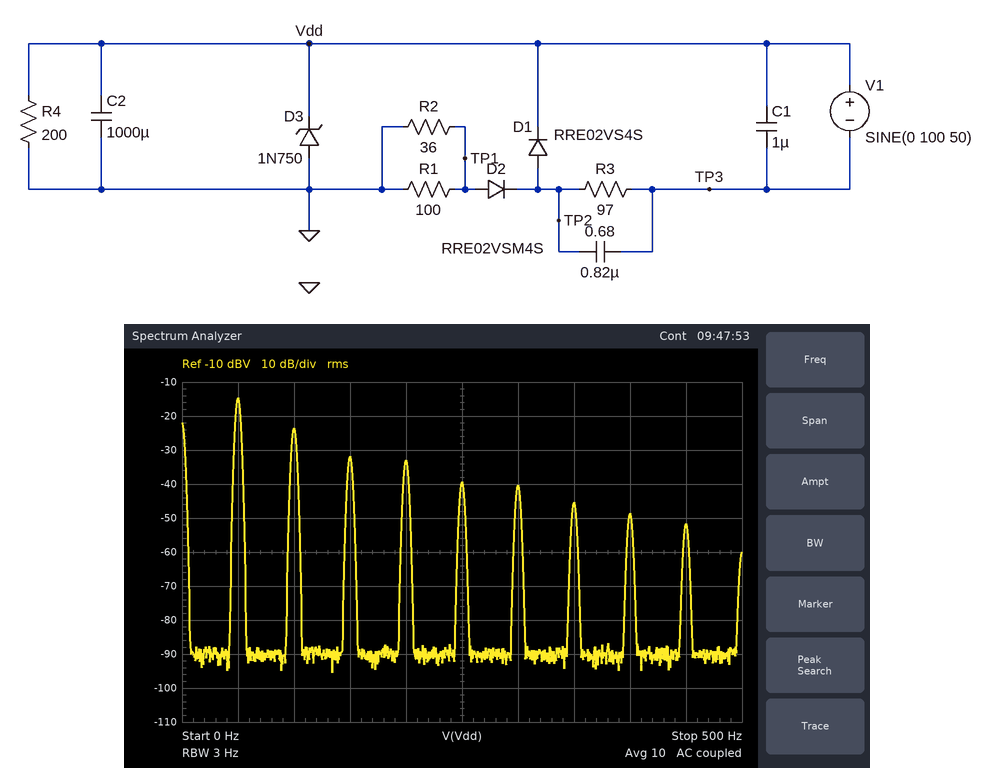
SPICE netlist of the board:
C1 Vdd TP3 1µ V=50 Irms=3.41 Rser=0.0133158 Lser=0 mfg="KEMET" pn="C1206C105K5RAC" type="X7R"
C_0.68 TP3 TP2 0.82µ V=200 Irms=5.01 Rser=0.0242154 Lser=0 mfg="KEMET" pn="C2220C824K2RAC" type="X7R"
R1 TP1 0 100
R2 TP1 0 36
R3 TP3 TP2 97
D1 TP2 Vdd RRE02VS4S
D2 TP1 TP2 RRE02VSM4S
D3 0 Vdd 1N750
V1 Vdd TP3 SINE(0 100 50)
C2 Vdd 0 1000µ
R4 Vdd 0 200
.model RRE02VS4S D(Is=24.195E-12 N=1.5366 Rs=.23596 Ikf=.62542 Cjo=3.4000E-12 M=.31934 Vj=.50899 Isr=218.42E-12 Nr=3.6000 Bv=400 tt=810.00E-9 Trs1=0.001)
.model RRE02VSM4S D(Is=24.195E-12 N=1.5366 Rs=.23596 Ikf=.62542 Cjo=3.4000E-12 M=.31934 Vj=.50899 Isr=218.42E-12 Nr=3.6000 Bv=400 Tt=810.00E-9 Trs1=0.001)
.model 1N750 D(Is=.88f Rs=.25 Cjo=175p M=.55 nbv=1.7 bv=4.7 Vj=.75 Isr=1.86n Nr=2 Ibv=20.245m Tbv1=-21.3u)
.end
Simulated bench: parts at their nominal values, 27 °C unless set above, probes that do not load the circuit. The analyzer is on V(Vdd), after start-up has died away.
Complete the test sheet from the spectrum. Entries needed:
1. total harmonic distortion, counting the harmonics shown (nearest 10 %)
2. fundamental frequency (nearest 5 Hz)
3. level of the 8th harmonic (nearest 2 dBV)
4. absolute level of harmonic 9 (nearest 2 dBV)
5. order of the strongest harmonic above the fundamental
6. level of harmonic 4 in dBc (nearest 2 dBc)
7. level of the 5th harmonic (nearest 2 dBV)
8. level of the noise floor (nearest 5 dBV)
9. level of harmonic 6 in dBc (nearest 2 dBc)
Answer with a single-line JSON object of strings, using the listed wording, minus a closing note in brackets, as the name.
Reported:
{"total harmonic distortion, counting the harmonics shown": "40 %", "fundamental frequency": "50 Hz", "level of the 8th harmonic": "-48 dBV", "absolute level of harmonic 9": "-52 dBV", "order of the strongest harmonic above the fundamental": "2", "level of harmonic 4 in dBc": "-18 dBc", "level of the 5th harmonic": "-40 dBV", "level of the noise floor": "-90 dBV", "level of harmonic 6 in dBc": "-26 dBc"}
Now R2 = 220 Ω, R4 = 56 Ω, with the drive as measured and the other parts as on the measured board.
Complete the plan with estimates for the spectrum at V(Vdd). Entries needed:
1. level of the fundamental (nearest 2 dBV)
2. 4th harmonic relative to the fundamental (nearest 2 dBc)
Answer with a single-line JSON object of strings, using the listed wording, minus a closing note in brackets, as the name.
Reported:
{"level of the fundamental": "-10 dBV", "4th harmonic relative to the fundamental": "-22 dBc"}
